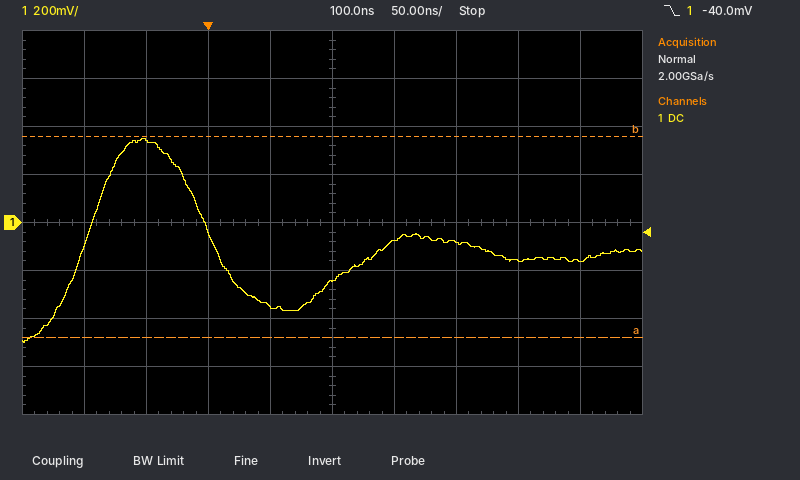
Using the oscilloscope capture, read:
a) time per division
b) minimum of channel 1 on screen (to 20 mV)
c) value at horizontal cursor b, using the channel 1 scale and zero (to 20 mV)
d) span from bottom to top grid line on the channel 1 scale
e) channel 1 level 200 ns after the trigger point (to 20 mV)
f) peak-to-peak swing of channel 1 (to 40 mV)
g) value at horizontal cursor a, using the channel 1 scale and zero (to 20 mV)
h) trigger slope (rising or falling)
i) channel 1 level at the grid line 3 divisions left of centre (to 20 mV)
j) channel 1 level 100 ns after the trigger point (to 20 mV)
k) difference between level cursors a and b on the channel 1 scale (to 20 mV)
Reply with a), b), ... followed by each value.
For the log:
a) 50 ns
b) -500 mV
c) 360 mV
d) 1.6 V
e) -80 mV
f) 840 mV
g) -480 mV
h) falling
i) 340 mV
j) -240 mV
k) 840 mV
